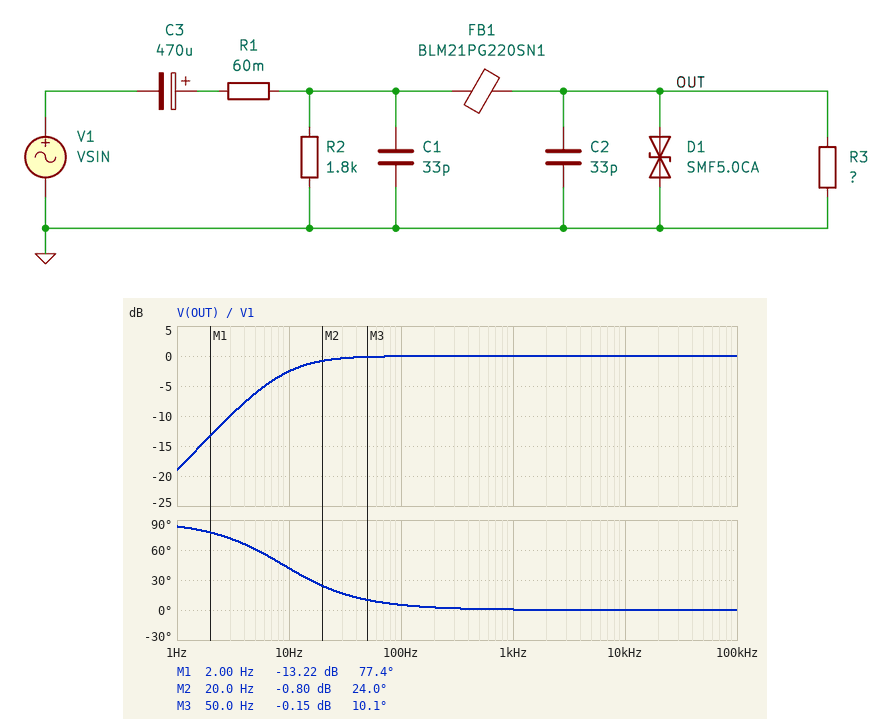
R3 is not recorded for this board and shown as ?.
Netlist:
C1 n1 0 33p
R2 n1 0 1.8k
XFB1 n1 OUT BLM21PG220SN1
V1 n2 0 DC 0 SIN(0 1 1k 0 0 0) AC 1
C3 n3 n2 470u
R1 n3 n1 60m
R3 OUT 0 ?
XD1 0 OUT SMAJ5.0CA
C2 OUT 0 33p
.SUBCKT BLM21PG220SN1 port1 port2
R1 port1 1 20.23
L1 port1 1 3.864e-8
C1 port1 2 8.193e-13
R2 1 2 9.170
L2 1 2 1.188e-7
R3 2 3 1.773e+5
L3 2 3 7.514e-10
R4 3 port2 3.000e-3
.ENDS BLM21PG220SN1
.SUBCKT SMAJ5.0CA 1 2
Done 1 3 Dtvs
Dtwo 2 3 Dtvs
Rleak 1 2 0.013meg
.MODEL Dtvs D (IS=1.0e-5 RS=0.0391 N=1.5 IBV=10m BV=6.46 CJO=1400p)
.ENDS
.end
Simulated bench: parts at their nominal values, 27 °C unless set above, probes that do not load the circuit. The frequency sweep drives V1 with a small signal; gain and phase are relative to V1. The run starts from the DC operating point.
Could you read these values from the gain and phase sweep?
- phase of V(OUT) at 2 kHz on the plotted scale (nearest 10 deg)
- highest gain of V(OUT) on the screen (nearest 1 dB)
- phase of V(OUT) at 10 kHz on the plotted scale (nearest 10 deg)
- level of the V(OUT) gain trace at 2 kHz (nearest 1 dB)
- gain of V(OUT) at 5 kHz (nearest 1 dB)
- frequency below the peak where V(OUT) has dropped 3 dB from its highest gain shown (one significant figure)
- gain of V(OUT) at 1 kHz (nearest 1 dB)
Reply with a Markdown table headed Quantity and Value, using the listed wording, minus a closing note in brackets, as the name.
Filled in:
| Quantity | Value |
|---|---|
| phase of V(OUT) at 2 kHz on the plotted scale | 0 deg |
| highest gain of V(OUT) on the screen | 0 dB |
| phase of V(OUT) at 10 kHz on the plotted scale | 0 deg |
| level of the V(OUT) gain trace at 2 kHz | 0 dB |
| gain of V(OUT) at 5 kHz | 0 dB |
| frequency below the peak where V(OUT) has dropped 3 dB from its highest gain shown | 9 Hz |
| gain of V(OUT) at 1 kHz | 0 dB |
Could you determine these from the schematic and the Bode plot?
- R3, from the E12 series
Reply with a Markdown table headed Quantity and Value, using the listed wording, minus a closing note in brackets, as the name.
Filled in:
| Quantity | Value |
|---|---|
| R3, from the E12 series | 39 Ω |
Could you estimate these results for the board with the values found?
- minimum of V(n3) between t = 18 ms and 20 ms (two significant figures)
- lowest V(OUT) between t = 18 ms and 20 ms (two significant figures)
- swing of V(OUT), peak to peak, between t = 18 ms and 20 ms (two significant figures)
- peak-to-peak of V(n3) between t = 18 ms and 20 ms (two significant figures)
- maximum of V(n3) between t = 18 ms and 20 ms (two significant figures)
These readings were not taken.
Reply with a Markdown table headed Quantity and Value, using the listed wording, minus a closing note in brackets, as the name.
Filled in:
| Quantity | Value |
|---|---|
| minimum of V(n3) between t = 18 ms and 20 ms | -1.0 V |
| lowest V(OUT) between t = 18 ms and 20 ms | -1.0 V |
| swing of V(OUT), peak to peak, between t = 18 ms and 20 ms | 2.0 V |
| peak-to-peak of V(n3) between t = 18 ms and 20 ms | 2.0 V |
| maximum of V(n3) between t = 18 ms and 20 ms | 1.0 V |
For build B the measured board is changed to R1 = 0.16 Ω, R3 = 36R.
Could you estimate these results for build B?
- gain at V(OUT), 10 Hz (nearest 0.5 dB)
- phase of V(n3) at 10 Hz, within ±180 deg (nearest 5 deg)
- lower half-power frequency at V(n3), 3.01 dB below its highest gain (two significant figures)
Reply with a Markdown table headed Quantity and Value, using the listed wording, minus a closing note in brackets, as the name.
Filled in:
| Quantity | Value |
|---|---|
| gain at V(OUT), 10 Hz | -3.0 dB |
| phase of V(n3) at 10 Hz, within ±180 deg | 45 deg |
| lower half-power frequency at V(n3), 3.01 dB below its highest gain | 9.6 Hz |
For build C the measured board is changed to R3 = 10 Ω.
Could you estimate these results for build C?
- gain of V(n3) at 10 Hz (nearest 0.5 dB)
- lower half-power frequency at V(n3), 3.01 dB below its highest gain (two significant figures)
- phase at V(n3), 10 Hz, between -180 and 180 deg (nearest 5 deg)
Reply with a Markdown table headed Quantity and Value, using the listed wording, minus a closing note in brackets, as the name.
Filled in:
| Quantity | Value |
|---|---|
| gain of V(n3) at 10 Hz | -11.0 dB |
| lower half-power frequency at V(n3), 3.01 dB below its highest gain | 34 Hz |
| phase at V(n3), 10 Hz, between -180 and 180 deg | 75 deg |
